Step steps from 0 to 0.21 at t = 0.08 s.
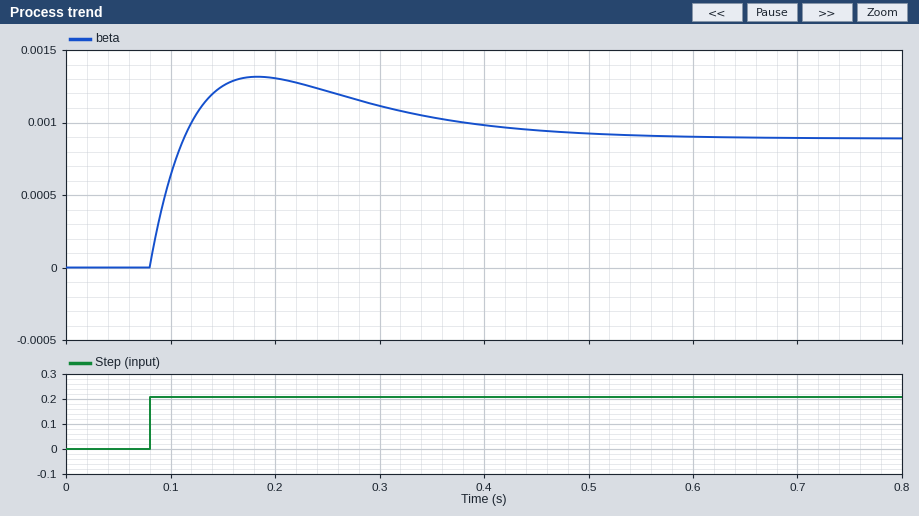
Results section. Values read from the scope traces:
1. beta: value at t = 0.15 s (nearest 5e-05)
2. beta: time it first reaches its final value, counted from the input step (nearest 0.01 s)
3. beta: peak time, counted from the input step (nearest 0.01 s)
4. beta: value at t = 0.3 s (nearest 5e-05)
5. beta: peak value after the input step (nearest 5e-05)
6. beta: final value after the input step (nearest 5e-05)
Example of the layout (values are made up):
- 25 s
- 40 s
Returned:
- 0.00125
- 0.03 s
- 0.10 s
- 0.00110
- 0.00130
- 0.00090
